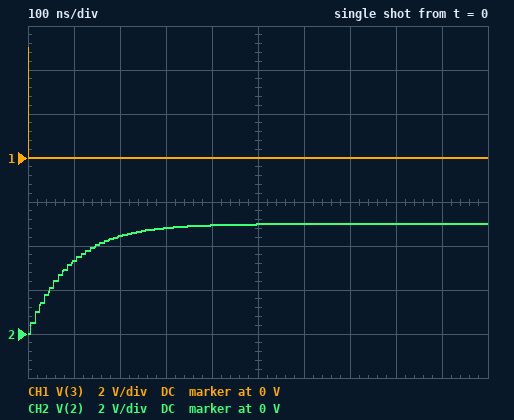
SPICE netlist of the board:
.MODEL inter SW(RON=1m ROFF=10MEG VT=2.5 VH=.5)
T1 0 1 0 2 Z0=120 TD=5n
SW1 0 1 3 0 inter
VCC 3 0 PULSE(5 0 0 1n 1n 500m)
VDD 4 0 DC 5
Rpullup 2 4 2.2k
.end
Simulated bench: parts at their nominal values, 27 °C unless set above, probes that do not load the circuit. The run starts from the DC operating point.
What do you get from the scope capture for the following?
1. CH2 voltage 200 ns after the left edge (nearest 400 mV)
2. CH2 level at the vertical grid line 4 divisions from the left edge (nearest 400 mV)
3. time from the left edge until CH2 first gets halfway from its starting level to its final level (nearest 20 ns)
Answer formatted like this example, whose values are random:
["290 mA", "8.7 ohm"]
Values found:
["4.4 V", "4.8 V", "60 ns"]
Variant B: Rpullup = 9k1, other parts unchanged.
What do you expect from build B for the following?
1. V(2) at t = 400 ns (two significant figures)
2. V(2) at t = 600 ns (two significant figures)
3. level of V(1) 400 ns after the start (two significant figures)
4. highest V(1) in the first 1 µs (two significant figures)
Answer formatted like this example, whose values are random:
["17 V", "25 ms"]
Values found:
["3.3 V", "4.0 V", "3.2 V", "4.6 V"]
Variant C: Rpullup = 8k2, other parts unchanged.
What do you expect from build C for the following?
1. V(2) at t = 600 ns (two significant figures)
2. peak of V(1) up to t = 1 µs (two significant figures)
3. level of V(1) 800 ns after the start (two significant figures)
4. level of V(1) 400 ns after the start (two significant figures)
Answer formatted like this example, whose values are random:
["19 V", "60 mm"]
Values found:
["4.1 V", "4.7 V", "4.5 V", "3.4 V"]
